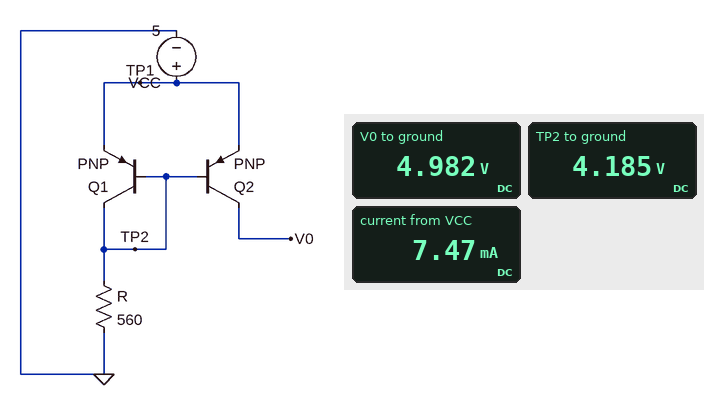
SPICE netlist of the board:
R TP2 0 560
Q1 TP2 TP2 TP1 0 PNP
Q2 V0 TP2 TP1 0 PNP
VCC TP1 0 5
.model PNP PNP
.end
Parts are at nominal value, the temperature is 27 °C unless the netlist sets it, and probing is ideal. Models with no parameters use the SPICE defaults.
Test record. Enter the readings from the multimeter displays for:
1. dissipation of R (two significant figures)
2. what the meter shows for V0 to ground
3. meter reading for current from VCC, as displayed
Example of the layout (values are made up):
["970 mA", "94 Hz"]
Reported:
["31 mW", "4.982 V", "7.47 mA"]
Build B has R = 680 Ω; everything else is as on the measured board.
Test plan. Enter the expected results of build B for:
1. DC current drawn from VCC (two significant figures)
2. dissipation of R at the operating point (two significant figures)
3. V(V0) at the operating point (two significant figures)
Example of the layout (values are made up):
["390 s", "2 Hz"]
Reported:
["6.2 mA", "26 mW", "5.0 V"]
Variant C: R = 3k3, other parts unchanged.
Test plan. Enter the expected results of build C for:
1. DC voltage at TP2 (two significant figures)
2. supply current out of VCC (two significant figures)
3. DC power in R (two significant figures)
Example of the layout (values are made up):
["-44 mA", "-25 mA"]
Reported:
["4.2 V", "1.3 mA", "5.4 mW"]
